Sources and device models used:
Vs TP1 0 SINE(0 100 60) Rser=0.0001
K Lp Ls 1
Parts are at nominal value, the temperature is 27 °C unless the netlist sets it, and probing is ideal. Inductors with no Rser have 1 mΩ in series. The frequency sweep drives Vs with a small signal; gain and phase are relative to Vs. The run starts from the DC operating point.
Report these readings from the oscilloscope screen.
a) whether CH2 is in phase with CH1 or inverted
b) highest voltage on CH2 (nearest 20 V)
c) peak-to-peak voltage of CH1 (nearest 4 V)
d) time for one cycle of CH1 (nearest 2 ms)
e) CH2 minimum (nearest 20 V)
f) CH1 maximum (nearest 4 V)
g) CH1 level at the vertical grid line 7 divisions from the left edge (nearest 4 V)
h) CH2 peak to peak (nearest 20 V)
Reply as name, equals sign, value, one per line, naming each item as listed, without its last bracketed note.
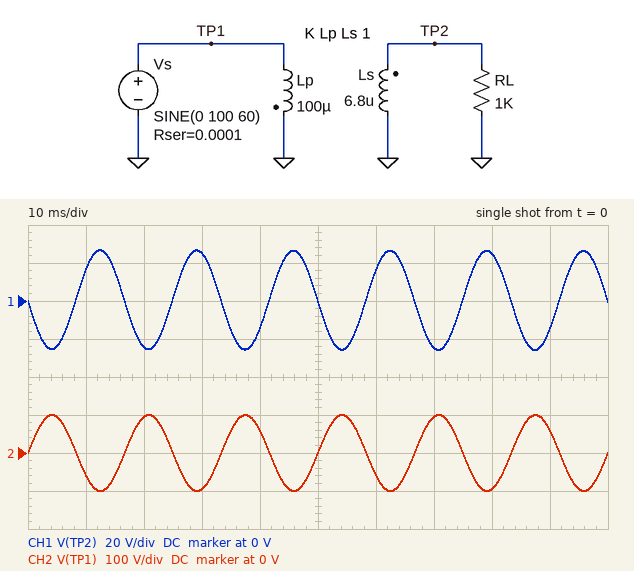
whether CH2 is in phase with CH1 or inverted = inverted
highest voltage on CH2 = 100 V
peak-to-peak voltage of CH1 = 52 V
time for one cycle of CH1 = 16 ms
CH2 minimum = -100 V
CH1 maximum = 28 V
CH1 level at the vertical grid line 7 divisions from the left edge = -24 V
CH2 peak to peak = 200 V
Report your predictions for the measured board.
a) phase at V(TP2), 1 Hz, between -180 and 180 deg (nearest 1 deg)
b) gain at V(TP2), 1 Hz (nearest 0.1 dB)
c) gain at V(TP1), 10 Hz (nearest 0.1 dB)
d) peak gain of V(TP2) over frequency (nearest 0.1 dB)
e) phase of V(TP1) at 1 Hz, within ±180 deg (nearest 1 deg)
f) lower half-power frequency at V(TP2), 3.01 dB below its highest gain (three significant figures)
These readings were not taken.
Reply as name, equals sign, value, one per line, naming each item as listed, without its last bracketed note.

phase at V(TP2), 1 Hz, between -180 and 180 deg = -120 deg
gain at V(TP2), 1 Hz = -17.8 dB
gain at V(TP1), 10 Hz = 0 dB
peak gain of V(TP2) over frequency = -11.7 dB
phase of V(TP1) at 1 Hz, within ±180 deg = 2 deg
lower half-power frequency at V(TP2), 3.01 dB below its highest gain = 1.75 Hz
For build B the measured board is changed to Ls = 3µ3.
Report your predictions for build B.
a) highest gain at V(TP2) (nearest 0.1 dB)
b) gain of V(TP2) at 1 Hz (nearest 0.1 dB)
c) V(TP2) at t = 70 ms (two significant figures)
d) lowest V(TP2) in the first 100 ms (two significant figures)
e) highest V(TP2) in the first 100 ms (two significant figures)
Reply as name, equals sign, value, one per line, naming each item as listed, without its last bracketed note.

highest gain at V(TP2) = -14.8 dB
gain of V(TP2) at 1 Hz = -20.9 dB
V(TP2) at t = 70 ms = -17 V
lowest V(TP2) in the first 100 ms = -18 V
highest V(TP2) in the first 100 ms = 19 V
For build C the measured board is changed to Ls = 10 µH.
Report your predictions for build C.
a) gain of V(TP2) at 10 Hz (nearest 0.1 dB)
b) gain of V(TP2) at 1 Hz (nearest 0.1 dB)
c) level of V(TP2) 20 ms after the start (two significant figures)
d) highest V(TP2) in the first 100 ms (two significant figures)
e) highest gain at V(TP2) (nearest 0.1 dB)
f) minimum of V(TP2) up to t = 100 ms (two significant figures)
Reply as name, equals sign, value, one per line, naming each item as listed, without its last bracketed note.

gain of V(TP2) at 10 Hz = -10.1 dB
gain of V(TP2) at 1 Hz = -16.1 dB
level of V(TP2) 20 ms after the start = -30 V
highest V(TP2) in the first 100 ms = 32 V
highest gain at V(TP2) = -10.0 dB
minimum of V(TP2) up to t = 100 ms = -31 V
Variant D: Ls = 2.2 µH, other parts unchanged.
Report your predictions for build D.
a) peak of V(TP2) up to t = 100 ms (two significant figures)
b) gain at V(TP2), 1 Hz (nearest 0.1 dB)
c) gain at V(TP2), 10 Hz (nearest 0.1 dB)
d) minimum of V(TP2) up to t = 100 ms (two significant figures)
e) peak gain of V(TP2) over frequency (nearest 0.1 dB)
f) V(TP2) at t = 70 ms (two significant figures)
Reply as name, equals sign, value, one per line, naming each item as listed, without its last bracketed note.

peak of V(TP2) up to t = 100 ms = 15 V
gain at V(TP2), 1 Hz = -22.7 dB
gain at V(TP2), 10 Hz = -16.7 dB
minimum of V(TP2) up to t = 100 ms = -15 V
peak gain of V(TP2) over frequency = -16.6 dB
V(TP2) at t = 70 ms = -14 V
